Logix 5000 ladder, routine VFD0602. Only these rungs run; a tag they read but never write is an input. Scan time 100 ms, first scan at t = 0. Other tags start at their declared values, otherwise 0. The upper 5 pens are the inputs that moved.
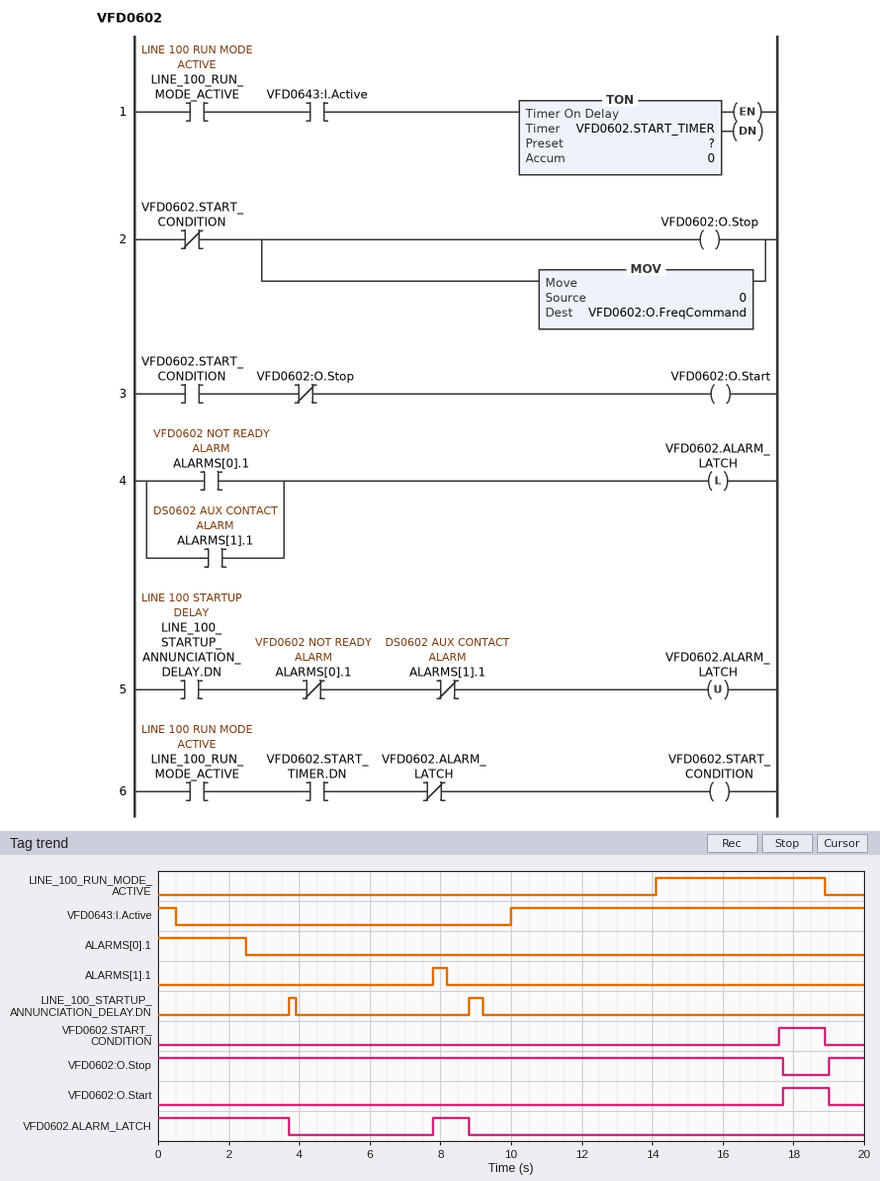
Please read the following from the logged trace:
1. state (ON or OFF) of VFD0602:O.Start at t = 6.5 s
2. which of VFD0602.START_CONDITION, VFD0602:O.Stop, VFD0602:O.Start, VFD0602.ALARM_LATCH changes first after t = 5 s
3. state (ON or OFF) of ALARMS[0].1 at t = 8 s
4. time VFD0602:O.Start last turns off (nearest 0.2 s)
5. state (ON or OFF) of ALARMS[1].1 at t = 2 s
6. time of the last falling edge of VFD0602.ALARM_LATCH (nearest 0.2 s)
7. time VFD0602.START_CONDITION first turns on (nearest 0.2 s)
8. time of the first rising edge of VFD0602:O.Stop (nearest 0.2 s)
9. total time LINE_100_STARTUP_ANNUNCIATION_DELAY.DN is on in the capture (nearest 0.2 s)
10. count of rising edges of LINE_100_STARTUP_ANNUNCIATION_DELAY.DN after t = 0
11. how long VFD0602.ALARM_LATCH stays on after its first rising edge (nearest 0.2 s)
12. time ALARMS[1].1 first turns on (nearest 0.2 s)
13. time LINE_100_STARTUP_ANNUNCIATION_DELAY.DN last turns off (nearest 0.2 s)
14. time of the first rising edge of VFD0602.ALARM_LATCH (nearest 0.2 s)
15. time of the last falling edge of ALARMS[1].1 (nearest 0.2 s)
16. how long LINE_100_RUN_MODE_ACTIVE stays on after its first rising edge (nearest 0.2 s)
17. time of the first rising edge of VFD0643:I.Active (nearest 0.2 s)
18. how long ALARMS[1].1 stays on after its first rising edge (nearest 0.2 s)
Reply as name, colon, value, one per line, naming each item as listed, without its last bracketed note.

state (ON or OFF) of VFD0602:O.Start at t = 6.5 s: OFF
which of VFD0602.START_CONDITION, VFD0602:O.Stop, VFD0602:O.Start, VFD0602.ALARM_LATCH changes first after t = 5 s: VFD0602.ALARM_LATCH
state (ON or OFF) of ALARMS[0].1 at t = 8 s: OFF
time VFD0602:O.Start last turns off: 19.0 s
state (ON or OFF) of ALARMS[1].1 at t = 2 s: OFF
time of the last falling edge of VFD0602.ALARM_LATCH: 8.8 s
time VFD0602.START_CONDITION first turns on: 17.6 s
time of the first rising edge of VFD0602:O.Stop: 19.0 s
total time LINE_100_STARTUP_ANNUNCIATION_DELAY.DN is on in the capture: 0.6 s
count of rising edges of LINE_100_STARTUP_ANNUNCIATION_DELAY.DN after t = 0: 2
how long VFD0602.ALARM_LATCH stays on after its first rising edge: 1.0 s
time ALARMS[1].1 first turns on: 7.8 s
time LINE_100_STARTUP_ANNUNCIATION_DELAY.DN last turns off: 9.2 s
time of the first rising edge of VFD0602.ALARM_LATCH: 7.8 s
time of the last falling edge of ALARMS[1].1: 8.2 s
how long LINE_100_RUN_MODE_ACTIVE stays on after its first rising edge: 4.8 s
time of the first rising edge of VFD0643:I.Active: 10.0 s
how long ALARMS[1].1 stays on after its first rising edge: 0.4 s
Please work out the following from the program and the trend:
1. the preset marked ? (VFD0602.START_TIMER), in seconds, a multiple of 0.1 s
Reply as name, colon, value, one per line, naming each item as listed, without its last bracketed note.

the preset marked ? (VFD0602.START_TIMER), in seconds, a multiple of 0.1 s: 3.5 s
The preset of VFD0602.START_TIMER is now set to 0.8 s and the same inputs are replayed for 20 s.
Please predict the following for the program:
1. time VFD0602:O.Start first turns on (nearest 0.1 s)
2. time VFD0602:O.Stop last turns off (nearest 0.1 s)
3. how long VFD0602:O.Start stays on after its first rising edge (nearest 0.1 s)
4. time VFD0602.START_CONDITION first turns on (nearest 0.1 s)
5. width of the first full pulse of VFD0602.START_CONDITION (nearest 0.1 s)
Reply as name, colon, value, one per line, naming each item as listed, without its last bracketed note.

time VFD0602:O.Start first turns on: 15.0 s
time VFD0602:O.Stop last turns off: 15.0 s
how long VFD0602:O.Start stays on after its first rising edge: 4.0 s
time VFD0602.START_CONDITION first turns on: 14.9 s
width of the first full pulse of VFD0602.START_CONDITION: 4.0 s
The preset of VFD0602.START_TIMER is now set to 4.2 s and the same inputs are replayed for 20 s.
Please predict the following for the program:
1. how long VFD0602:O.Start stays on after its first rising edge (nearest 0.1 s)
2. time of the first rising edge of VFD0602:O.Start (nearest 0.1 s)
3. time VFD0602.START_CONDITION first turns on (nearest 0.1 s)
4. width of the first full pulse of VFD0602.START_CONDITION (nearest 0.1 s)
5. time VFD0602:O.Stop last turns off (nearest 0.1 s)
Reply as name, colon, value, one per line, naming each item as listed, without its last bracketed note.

how long VFD0602:O.Start stays on after its first rising edge: 0.6 s
time of the first rising edge of VFD0602:O.Start: 18.4 s
time VFD0602.START_CONDITION first turns on: 18.3 s
width of the first full pulse of VFD0602.START_CONDITION: 0.6 s
time VFD0602:O.Stop last turns off: 18.4 s
